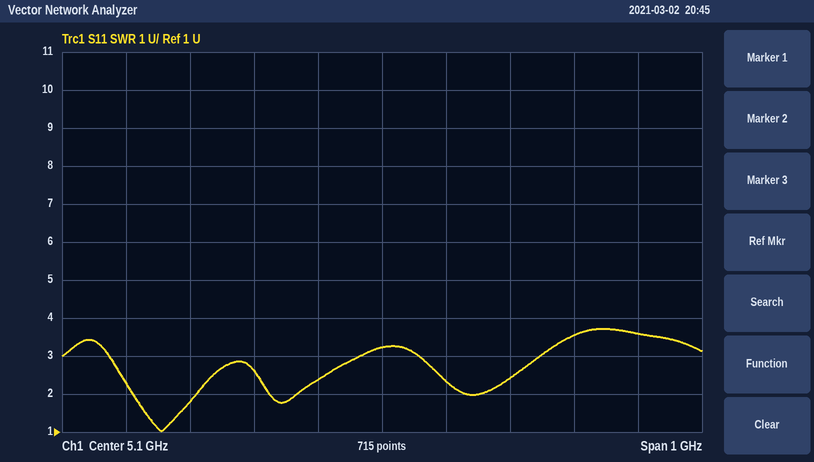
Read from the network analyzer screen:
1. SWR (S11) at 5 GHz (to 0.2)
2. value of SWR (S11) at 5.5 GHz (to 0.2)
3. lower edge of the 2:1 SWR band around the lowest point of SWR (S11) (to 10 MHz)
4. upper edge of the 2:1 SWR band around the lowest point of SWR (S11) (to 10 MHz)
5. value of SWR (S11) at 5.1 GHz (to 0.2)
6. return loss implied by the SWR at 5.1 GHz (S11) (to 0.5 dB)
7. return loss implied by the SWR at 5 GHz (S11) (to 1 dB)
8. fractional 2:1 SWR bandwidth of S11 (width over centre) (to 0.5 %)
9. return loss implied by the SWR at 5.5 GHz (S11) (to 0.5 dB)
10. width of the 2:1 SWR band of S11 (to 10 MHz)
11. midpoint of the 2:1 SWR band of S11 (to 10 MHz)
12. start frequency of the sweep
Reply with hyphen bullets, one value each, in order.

- 2.4
- 3.6
- 4.71 GHz
- 4.81 GHz
- 3.2
- 5.5 dB
- 8 dB
- 2.0 %
- 5.0 dB
- 100 MHz
- 4.76 GHz
- 4.6 GHz
